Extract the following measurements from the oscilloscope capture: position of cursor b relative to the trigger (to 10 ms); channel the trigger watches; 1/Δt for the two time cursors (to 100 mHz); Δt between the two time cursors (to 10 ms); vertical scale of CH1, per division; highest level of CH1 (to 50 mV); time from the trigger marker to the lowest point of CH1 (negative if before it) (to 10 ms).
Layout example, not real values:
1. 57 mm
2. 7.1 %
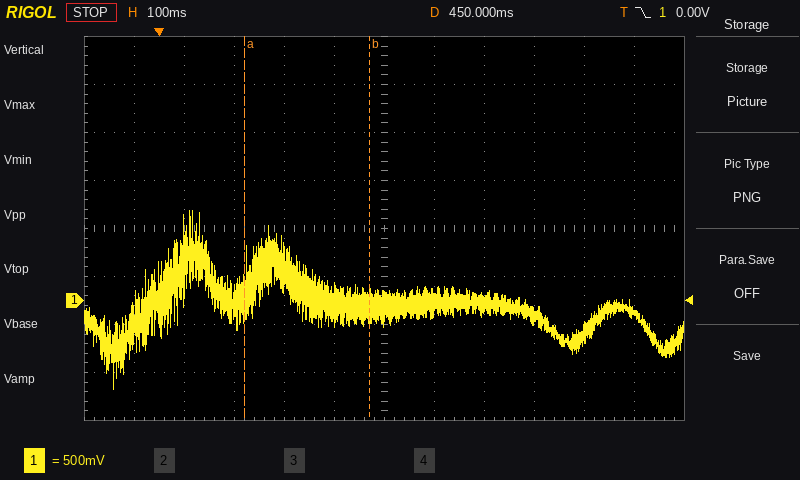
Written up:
1. +420 ms
2. CH1
3. 4.0 Hz
4. 250 ms
5. 500 mV
6. 950 mV
7. -90 ms
